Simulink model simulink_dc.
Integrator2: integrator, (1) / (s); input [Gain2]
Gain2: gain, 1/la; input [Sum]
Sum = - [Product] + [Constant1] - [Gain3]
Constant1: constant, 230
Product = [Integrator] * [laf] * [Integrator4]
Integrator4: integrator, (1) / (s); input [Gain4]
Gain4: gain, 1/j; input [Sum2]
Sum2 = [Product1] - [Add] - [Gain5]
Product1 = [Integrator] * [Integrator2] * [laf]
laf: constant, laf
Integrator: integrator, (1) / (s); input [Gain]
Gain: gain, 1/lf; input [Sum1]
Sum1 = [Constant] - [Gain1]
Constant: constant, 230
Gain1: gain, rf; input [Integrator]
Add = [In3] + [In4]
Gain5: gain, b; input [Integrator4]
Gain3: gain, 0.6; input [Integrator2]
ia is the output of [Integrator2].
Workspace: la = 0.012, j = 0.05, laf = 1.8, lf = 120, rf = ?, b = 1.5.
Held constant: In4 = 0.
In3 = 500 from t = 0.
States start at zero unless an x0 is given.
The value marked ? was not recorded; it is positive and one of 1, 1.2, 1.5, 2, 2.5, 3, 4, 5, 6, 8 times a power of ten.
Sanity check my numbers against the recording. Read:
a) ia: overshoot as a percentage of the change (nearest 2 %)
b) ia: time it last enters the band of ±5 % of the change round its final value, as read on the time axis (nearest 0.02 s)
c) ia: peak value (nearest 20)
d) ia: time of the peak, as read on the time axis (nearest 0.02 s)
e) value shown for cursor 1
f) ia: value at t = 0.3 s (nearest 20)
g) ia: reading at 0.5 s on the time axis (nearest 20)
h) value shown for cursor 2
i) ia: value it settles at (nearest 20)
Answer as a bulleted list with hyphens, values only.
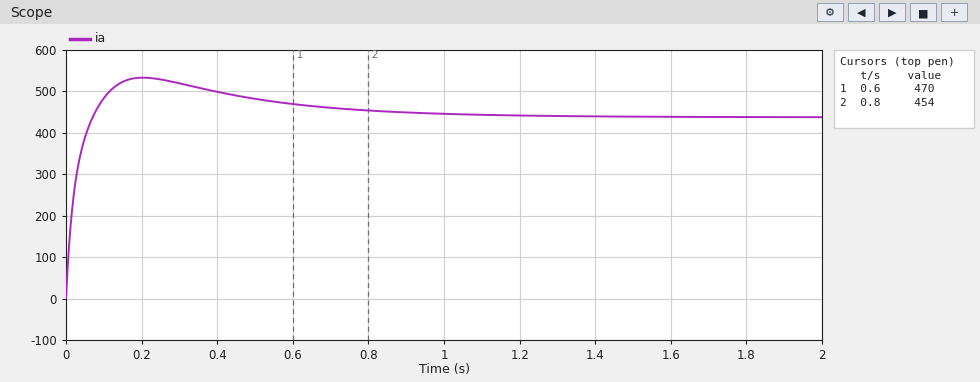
- 22 %
- 0.72 s
- 540
- 0.20 s
- 470
- 520
- 480
- 454
- 440
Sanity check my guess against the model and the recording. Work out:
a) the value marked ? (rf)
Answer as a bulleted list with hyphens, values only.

- 400
